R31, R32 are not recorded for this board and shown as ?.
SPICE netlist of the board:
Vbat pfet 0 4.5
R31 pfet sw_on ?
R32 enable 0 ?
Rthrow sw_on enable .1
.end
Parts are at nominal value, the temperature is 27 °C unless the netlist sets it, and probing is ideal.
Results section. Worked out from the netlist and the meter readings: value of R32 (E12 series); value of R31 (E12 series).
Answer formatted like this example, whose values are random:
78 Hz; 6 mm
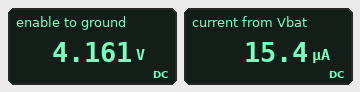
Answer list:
270 kΩ; 22 kΩ
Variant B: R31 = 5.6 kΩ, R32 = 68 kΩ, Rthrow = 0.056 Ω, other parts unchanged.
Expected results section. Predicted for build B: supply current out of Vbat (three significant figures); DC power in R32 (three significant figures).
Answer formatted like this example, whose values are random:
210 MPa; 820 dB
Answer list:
61.1 µA; 254 µW
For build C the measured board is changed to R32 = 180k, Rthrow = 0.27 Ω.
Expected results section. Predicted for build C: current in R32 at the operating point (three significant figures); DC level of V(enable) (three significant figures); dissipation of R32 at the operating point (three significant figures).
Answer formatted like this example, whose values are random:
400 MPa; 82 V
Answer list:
22.3 µA; 4.01 V; 89.3 µW
